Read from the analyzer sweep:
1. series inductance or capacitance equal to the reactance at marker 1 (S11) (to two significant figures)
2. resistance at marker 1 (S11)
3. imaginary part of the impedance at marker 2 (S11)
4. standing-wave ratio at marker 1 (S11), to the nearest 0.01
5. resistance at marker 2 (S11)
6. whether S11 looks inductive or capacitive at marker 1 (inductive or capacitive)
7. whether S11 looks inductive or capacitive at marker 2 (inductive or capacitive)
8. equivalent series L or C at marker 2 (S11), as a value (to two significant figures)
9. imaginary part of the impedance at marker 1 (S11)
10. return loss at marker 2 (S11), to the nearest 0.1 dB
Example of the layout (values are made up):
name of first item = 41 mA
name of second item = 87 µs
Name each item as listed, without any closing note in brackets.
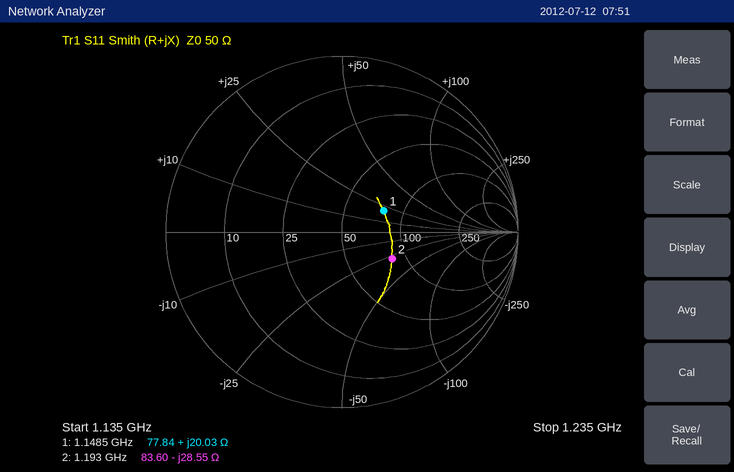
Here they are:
series inductance or capacitance equal to the reactance at marker 1 (S11) = 2.8 nH
resistance at marker 1 = 77.84 Ω
imaginary part of the impedance at marker 2 = -28.55 Ω
standing-wave ratio at marker 1 (S11), to the nearest 0.01 = 1.72
resistance at marker 2 = 83.60 Ω
whether S11 looks inductive or capacitive at marker 1 = inductive
whether S11 looks inductive or capacitive at marker 2 = capacitive
equivalent series L or C at marker 2 (S11), as a value = 4.7 pF
imaginary part of the impedance at marker 1 = +20.03 Ω
return loss at marker 2 (S11), to the nearest 0.1 dB = 9.8 dB
